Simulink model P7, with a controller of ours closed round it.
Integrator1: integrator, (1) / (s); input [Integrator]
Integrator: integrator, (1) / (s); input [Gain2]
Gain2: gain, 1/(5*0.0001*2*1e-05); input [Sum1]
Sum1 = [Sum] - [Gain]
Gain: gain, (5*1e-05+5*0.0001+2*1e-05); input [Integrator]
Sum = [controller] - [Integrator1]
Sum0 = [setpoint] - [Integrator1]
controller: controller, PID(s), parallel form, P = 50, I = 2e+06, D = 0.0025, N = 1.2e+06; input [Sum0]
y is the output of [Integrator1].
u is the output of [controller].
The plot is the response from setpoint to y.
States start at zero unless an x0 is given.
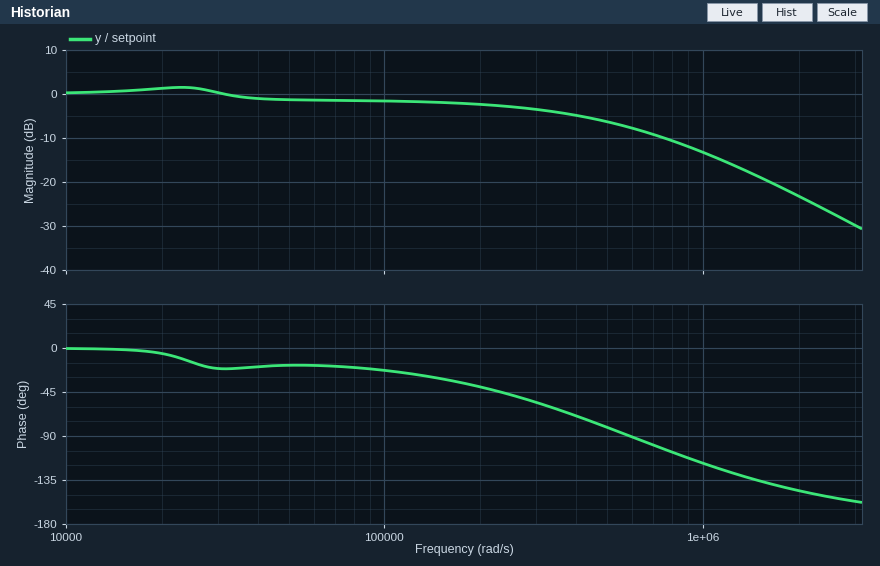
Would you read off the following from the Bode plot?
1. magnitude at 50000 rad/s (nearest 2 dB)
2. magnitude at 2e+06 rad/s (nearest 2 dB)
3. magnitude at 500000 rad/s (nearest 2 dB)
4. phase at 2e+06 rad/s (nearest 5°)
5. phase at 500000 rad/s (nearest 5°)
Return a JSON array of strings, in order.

["-2 dB", "-24 dB", "-6 dB", "-145°", "-80°"]
